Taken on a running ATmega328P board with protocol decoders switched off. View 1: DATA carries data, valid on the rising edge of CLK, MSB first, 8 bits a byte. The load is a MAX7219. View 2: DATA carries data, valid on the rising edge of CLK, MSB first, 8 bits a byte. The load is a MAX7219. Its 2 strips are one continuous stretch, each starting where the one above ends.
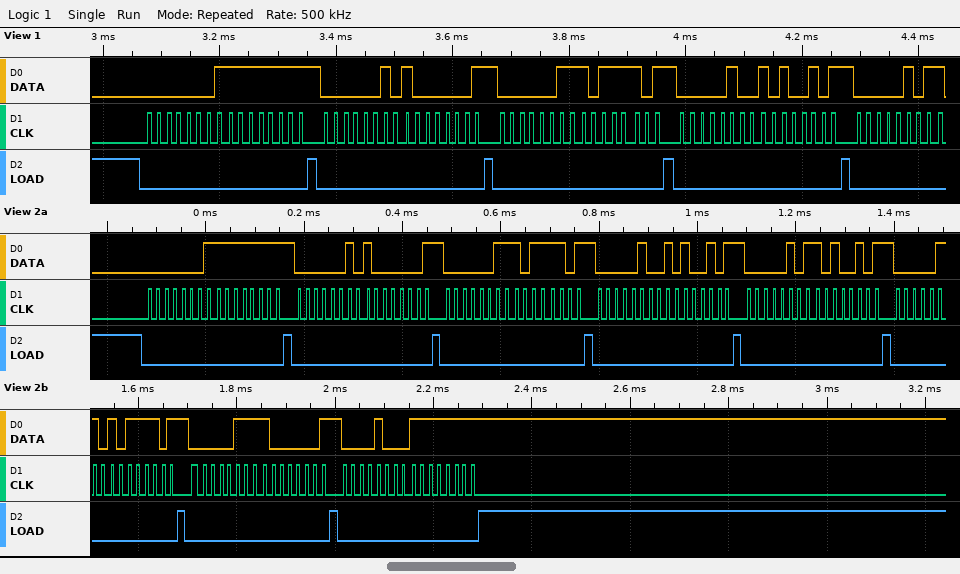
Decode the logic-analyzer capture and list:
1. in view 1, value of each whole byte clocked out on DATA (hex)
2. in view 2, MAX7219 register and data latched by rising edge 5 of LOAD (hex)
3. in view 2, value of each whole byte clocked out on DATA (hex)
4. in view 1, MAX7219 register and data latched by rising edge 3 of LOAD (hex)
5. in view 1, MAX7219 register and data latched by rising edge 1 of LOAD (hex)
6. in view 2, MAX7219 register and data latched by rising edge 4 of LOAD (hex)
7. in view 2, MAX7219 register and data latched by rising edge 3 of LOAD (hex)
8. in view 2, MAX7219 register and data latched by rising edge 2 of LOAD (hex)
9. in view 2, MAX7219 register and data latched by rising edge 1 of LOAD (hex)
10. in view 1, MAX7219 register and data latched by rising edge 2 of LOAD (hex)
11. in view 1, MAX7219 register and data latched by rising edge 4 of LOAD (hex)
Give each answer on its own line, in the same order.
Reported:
01 FF 02 81 03 BD 04 A5 05
register 0x5, data 0xA5
0x01 0xFF 0x02 0x81 0x03 0xBD 0x04 0xA5 0x05 0xA5 0x06 0xBD 0x07 0x81 0x08 0xFF
register 0x3, data 0xBD
register 0x1, data 0xFF
register 0x4, data 0xA5
register 0x3, data 0xBD
register 0x2, data 0x81
register 0x1, data 0xFF
register 0x2, data 0x81
register 0x4, data 0xA5
